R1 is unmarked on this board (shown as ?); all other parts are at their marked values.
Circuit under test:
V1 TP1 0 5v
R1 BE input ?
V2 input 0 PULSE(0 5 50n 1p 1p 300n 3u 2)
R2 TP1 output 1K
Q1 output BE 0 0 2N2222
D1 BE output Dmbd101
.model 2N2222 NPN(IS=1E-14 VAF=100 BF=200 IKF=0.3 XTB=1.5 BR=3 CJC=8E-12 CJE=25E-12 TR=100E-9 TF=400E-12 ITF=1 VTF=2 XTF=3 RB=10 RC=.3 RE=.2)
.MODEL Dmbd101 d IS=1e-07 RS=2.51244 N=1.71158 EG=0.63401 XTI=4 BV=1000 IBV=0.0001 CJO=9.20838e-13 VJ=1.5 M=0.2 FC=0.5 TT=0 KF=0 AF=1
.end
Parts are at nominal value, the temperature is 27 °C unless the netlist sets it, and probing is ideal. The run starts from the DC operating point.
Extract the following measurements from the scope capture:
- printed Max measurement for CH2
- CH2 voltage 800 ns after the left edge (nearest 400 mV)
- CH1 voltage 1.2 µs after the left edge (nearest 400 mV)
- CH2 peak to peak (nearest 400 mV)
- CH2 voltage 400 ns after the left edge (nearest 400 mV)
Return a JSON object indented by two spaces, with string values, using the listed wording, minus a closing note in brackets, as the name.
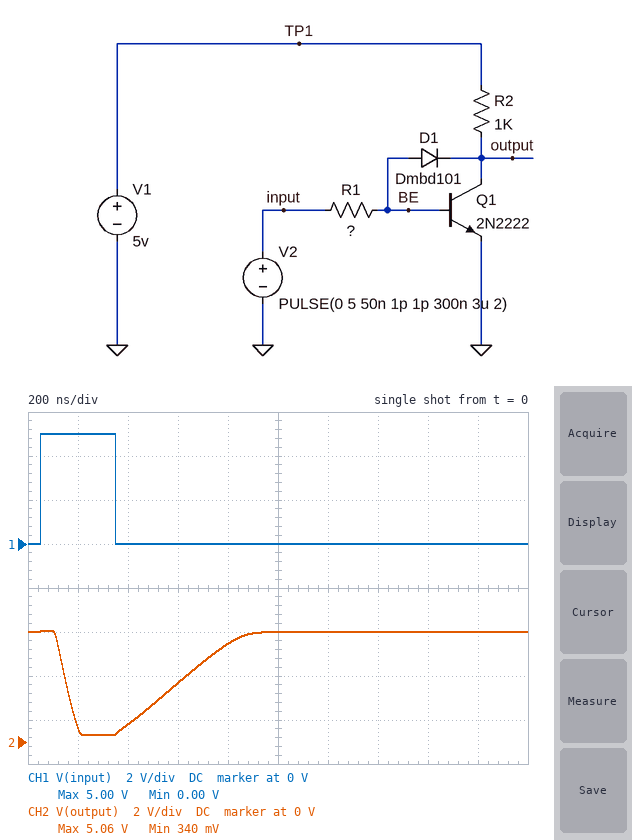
{
  "printed Max measurement for CH2": "5.06 V",
  "CH2 voltage 800 ns after the left edge": "4.4 V",
  "CH1 voltage 1.2 µs after the left edge": "0 V",
  "CH2 peak to peak": "4.8 V",
  "CH2 voltage 400 ns after the left edge": "800 mV"
}
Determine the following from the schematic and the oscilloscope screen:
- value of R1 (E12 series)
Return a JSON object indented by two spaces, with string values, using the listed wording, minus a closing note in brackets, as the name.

{
  "value of R1": "12 kΩ"
}
